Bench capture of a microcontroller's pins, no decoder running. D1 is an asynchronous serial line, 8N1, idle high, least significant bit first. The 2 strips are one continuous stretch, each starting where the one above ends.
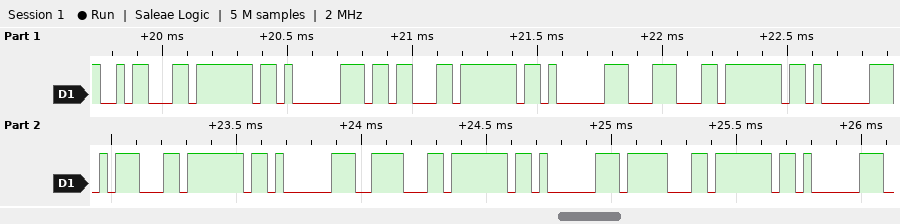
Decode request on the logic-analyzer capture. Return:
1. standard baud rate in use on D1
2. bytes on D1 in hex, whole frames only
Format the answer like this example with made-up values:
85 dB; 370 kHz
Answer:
31250 baud; 1A 7F 81 1B 7F 81 1C 7F 81 1D 7F 81 1E 7F 81 1F 7F 81
